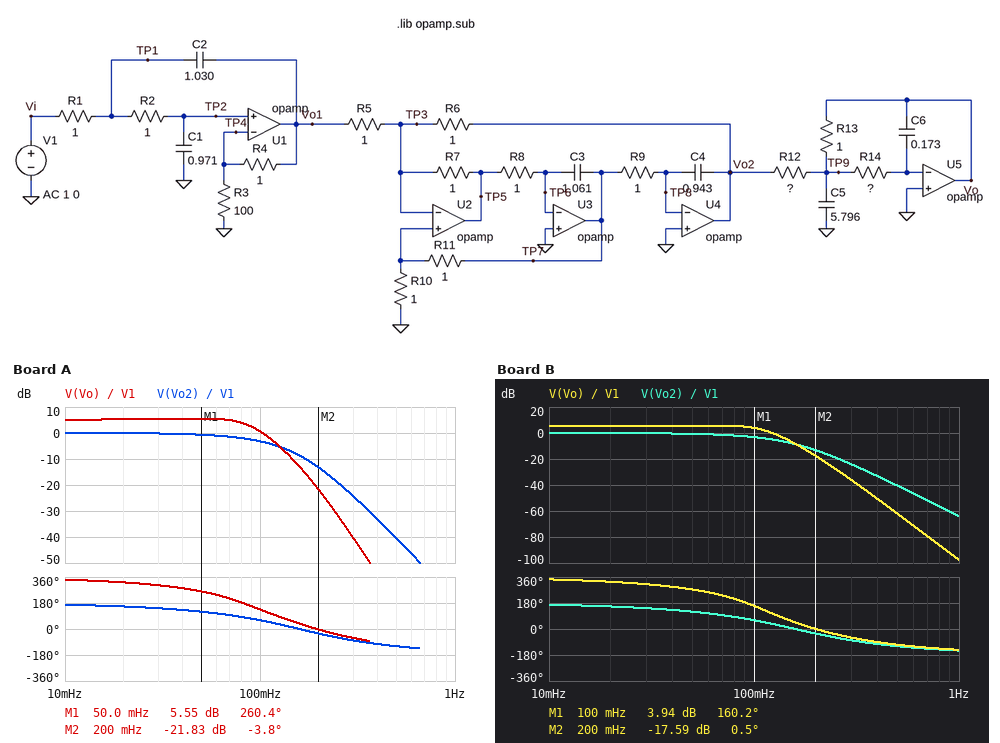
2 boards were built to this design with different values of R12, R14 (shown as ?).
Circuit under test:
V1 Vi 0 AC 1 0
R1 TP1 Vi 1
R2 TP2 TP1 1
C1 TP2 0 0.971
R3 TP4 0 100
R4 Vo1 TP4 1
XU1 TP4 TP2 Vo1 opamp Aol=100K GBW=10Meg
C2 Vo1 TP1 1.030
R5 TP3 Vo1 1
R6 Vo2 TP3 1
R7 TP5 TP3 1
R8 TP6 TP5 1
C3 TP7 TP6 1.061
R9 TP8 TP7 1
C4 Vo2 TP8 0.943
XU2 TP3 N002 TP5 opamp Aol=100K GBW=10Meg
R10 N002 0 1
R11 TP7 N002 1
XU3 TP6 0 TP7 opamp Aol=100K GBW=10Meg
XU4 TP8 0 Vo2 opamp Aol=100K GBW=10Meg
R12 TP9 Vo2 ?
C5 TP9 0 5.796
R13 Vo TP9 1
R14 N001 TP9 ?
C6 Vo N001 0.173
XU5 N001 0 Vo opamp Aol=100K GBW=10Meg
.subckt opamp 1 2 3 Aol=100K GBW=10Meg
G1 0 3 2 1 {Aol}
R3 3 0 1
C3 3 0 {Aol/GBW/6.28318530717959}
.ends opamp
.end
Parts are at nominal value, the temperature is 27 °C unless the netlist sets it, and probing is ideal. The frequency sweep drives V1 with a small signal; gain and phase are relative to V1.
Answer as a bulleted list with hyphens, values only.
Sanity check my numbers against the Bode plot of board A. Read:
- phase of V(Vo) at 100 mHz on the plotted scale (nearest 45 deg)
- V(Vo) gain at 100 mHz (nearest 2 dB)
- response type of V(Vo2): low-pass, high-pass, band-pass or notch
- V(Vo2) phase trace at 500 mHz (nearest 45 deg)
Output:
- 135 deg
- 0 dB
- low-pass
- -135 deg
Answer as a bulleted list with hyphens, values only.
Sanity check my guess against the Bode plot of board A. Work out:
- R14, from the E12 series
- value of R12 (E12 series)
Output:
- 3.3 Ω
- 0.56 Ω
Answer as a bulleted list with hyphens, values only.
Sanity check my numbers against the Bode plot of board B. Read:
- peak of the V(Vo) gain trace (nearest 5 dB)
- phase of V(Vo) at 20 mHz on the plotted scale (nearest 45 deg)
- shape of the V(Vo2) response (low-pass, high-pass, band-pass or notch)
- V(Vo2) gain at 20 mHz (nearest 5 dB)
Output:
- 5 dB
- 315 deg
- low-pass
- 0 dB
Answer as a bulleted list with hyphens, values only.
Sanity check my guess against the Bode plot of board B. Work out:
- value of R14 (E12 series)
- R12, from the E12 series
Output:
- 2.2 Ω
- 0.56 Ω
